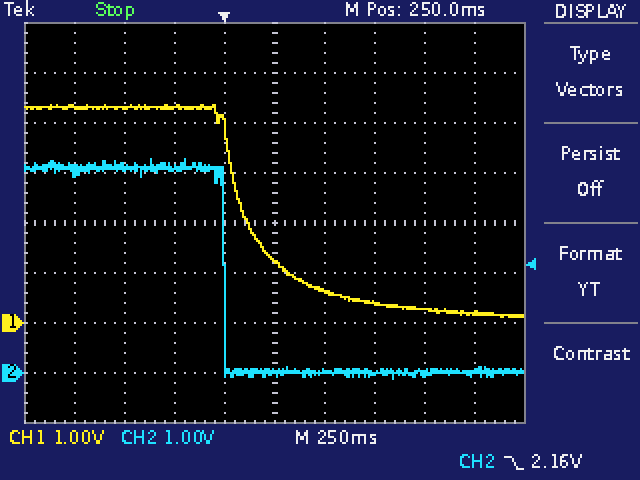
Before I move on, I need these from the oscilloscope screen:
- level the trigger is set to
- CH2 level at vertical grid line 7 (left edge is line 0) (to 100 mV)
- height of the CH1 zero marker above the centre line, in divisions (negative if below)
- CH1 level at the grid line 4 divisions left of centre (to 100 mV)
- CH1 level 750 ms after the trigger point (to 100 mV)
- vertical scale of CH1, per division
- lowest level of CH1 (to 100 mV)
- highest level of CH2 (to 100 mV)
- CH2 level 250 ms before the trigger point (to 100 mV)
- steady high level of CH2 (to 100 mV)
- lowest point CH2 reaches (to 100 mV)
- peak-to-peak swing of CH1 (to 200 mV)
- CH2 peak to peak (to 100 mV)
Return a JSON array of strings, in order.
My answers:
["2.16 V", "0.0 V", "-2.0 div", "4.3 V", "400 mV", "1 V", "100 mV", "4.3 V", "4.1 V", "4.1 V", "-100 mV", "4.2 V", "4.4 V"]
